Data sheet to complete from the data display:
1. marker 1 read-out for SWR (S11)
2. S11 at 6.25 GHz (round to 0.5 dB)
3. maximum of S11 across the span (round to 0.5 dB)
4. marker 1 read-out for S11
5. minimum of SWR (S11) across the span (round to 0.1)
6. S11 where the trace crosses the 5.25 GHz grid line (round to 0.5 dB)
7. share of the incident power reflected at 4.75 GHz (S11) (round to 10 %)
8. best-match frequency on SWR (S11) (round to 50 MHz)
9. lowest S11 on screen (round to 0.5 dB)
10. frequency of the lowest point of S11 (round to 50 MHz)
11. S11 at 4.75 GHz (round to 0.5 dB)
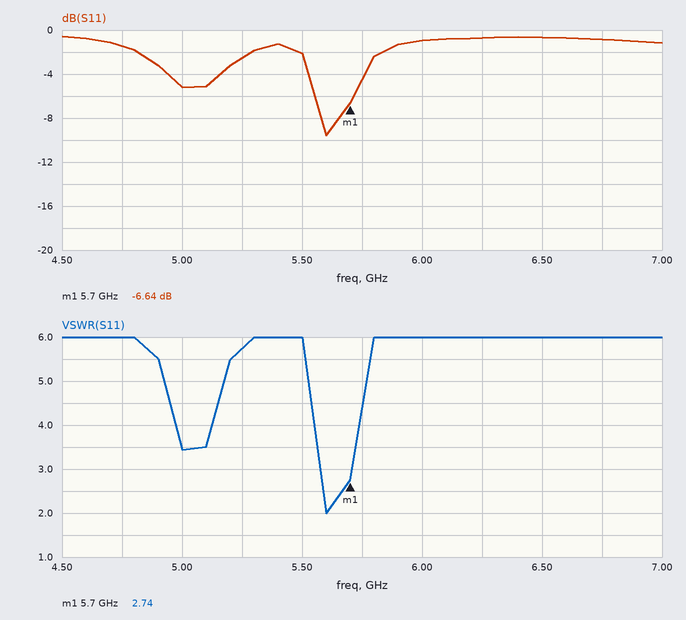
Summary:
2.74
-0.5 dB
-0.5 dB
-6.64 dB
2.0
-2.5 dB
70 %
5.60 GHz
-9.5 dB
5.60 GHz
-1.5 dB
